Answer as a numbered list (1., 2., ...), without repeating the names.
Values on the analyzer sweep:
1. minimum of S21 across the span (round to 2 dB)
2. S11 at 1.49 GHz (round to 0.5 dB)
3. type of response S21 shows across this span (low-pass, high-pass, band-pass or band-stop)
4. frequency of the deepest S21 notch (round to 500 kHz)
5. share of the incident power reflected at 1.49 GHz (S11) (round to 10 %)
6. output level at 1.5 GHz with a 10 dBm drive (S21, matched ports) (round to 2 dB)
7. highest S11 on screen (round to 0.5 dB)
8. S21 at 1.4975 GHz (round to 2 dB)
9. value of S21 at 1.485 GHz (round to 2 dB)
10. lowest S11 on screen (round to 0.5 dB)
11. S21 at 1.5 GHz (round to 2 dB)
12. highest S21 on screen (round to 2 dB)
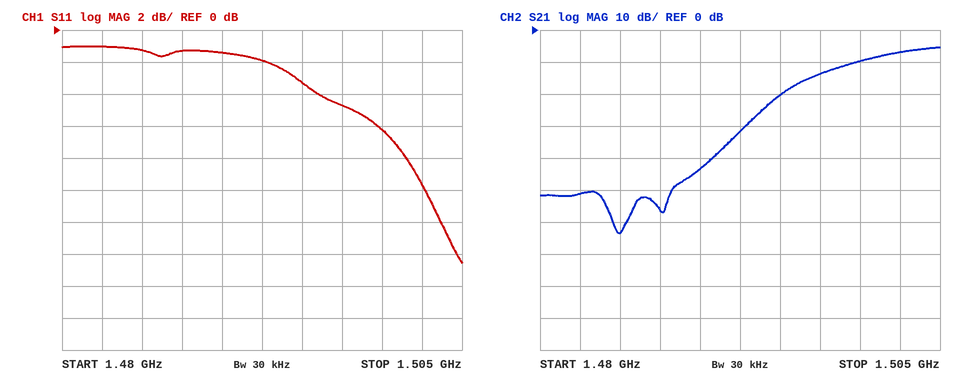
1. -64 dB
2. -1.5 dB
3. high-pass
4. 1.4850 GHz
5. 70 %
6. 0 dBm
7. -1.0 dB
8. -14 dB
9. -64 dB
10. -14.5 dB
11. -10 dB
12. -6 dB
